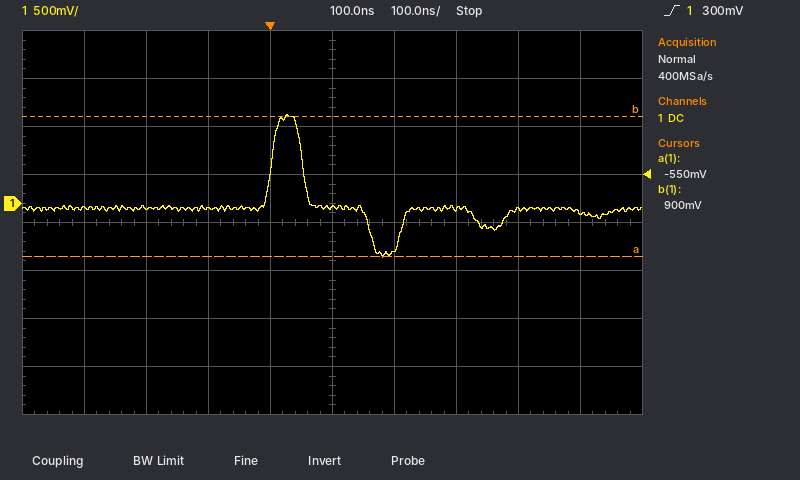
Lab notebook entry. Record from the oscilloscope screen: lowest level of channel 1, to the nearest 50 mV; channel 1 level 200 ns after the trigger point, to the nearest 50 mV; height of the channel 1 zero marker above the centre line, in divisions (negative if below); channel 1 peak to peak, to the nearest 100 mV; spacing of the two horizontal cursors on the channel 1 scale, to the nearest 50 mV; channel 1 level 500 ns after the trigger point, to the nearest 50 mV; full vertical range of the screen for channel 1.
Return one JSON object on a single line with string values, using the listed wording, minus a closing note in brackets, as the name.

{"lowest level of channel 1, to the nearest 50 mV": "-550 mV", "channel 1 level 200 ns after the trigger point, to the nearest 50 mV": "-500 mV", "height of the channel 1 zero marker above the centre line, in divisions": "+0.4 div", "channel 1 peak to peak, to the nearest 100 mV": "1.50 V", "spacing of the two horizontal cursors on the channel 1 scale, to the nearest 50 mV": "1.45 V", "channel 1 level 500 ns after the trigger point, to the nearest 50 mV": "-100 mV", "full vertical range of the screen for channel 1": "4 V"}
